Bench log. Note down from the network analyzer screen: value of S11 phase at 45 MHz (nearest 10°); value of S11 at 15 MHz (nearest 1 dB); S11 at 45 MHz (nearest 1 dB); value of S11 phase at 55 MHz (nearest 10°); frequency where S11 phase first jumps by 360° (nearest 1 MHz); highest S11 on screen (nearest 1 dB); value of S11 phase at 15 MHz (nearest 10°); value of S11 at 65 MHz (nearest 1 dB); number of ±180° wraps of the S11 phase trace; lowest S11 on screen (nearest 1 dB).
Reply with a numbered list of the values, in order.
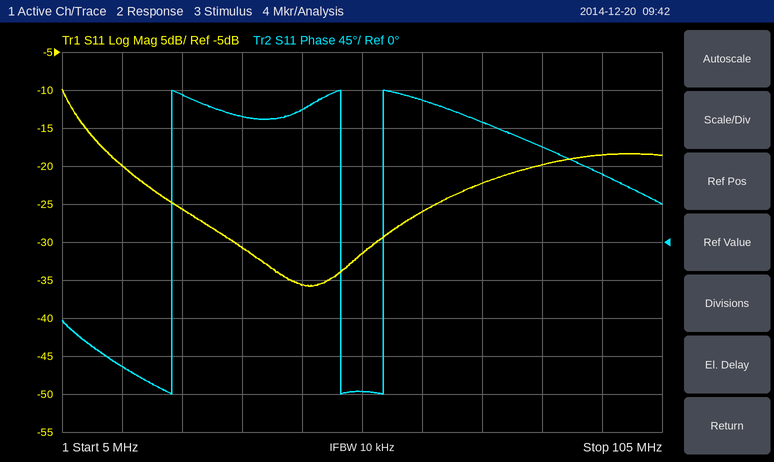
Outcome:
1. 160°
2. -20 dB
3. -36 dB
4. -180°
5. 23 MHz
6. -10 dB
7. -150°
8. -26 dB
9. 3
10. -36 dB
